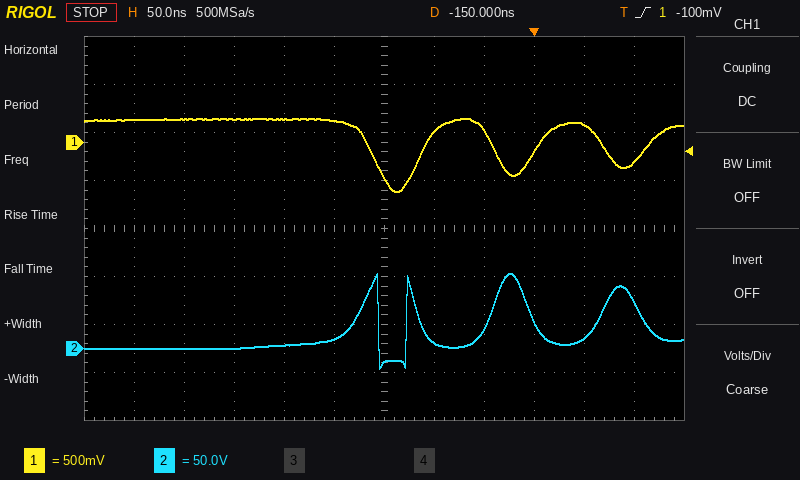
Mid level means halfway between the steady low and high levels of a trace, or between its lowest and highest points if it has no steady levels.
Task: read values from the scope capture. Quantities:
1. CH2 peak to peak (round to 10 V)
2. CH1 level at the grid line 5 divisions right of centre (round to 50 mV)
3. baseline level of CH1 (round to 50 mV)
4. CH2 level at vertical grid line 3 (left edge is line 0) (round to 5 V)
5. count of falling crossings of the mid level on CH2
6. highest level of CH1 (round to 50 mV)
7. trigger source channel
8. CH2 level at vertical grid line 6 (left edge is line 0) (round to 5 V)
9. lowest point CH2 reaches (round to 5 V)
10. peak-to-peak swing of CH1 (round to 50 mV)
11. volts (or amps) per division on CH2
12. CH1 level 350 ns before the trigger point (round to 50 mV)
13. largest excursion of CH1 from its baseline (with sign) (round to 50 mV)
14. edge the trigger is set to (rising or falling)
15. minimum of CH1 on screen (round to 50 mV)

100 V
-200 mV
250 mV
0 V
4
250 mV
CH1
-15 V
-20 V
750 mV
50 V
250 mV
-750 mV
rising
-500 mV
